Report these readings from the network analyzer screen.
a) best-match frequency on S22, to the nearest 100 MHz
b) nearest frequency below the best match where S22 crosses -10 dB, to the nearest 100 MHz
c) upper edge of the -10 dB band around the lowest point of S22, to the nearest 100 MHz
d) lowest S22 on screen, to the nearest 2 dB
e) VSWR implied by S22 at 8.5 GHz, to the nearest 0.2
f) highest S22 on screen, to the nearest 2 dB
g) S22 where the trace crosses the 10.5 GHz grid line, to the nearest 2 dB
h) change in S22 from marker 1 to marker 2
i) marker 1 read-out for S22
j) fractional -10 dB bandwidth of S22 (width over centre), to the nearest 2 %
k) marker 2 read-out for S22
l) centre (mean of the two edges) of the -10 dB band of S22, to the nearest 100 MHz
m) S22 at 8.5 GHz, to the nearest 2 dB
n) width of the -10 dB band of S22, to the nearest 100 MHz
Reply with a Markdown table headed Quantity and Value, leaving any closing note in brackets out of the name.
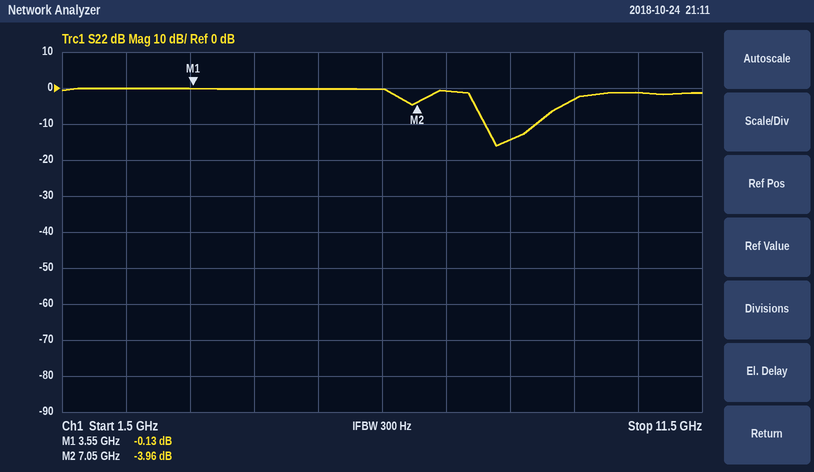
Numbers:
| Quantity | Value |
|---|---|
| best-match frequency on S22, to the nearest 100 MHz | 8.3 GHz |
| nearest frequency below the best match where S22 crosses -10 dB, to the nearest 100 MHz | 8.1 GHz |
| upper edge of the -10 dB band around the lowest point of S22, to the nearest 100 MHz | 8.9 GHz |
| lowest S22 on screen, to the nearest 2 dB | -16 dB |
| VSWR implied by S22 at 8.5 GHz, to the nearest 0.2 | 1.4 |
| highest S22 on screen, to the nearest 2 dB | 0 dB |
| S22 where the trace crosses the 10.5 GHz grid line, to the nearest 2 dB | -2 dB |
| change in S22 from marker 1 to marker 2 | -3.83 dB |
| marker 1 read-out for S22 | -0.13 dB |
| fractional -10 dB bandwidth of S22 (width over centre), to the nearest 2 % | 10 % |
| marker 2 read-out for S22 | -3.96 dB |
| centre (mean of the two edges) of the -10 dB band of S22, to the nearest 100 MHz | 8.5 GHz |
| S22 at 8.5 GHz, to the nearest 2 dB | -14 dB |
| width of the -10 dB band of S22, to the nearest 100 MHz | 800 MHz |
